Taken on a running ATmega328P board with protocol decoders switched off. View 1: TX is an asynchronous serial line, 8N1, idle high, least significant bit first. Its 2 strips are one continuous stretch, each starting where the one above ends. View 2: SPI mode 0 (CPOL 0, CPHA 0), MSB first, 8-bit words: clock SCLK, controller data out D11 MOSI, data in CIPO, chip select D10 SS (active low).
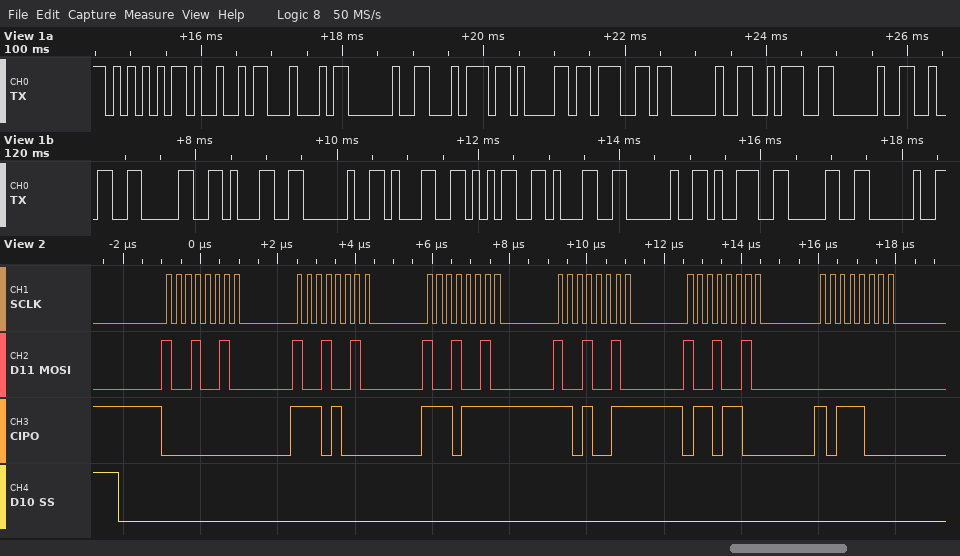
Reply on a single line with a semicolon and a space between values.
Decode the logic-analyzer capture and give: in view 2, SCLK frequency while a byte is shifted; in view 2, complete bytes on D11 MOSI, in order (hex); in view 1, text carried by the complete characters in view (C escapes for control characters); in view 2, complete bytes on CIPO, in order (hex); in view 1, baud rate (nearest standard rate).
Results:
4 MHz; 92 92 92 92 92 00; "UID tag : 201 151 90 "; 00 E8 EF D3 6C B8; 9600 baud
